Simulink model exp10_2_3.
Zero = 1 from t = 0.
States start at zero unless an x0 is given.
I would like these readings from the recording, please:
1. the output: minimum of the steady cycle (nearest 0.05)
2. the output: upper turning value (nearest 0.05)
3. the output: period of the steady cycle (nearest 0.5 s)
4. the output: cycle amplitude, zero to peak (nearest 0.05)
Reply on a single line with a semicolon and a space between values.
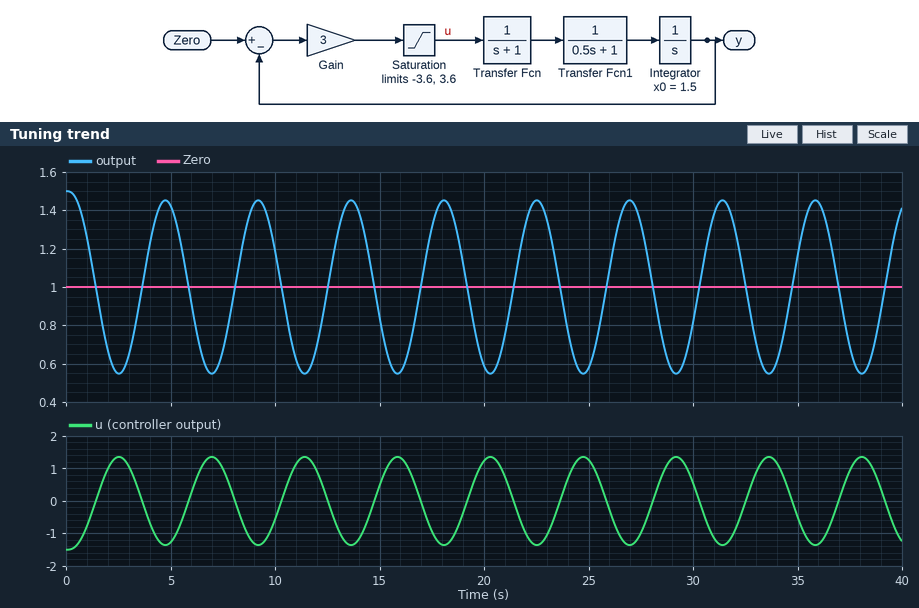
0.55; 1.45; 4.5 s; 0.45
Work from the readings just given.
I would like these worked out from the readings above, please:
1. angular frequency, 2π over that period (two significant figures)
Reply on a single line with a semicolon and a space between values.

1.4 rad/s
